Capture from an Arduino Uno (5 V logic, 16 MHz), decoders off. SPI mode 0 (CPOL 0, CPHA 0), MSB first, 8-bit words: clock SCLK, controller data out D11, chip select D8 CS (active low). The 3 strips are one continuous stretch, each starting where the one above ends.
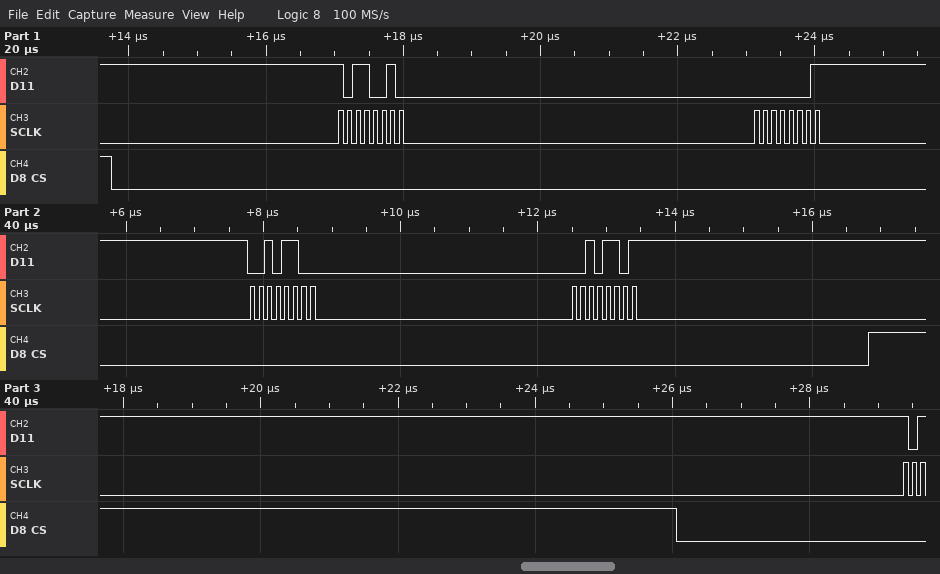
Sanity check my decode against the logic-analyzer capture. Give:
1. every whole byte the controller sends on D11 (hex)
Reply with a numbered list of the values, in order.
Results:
1. B2 01 2C 2D
